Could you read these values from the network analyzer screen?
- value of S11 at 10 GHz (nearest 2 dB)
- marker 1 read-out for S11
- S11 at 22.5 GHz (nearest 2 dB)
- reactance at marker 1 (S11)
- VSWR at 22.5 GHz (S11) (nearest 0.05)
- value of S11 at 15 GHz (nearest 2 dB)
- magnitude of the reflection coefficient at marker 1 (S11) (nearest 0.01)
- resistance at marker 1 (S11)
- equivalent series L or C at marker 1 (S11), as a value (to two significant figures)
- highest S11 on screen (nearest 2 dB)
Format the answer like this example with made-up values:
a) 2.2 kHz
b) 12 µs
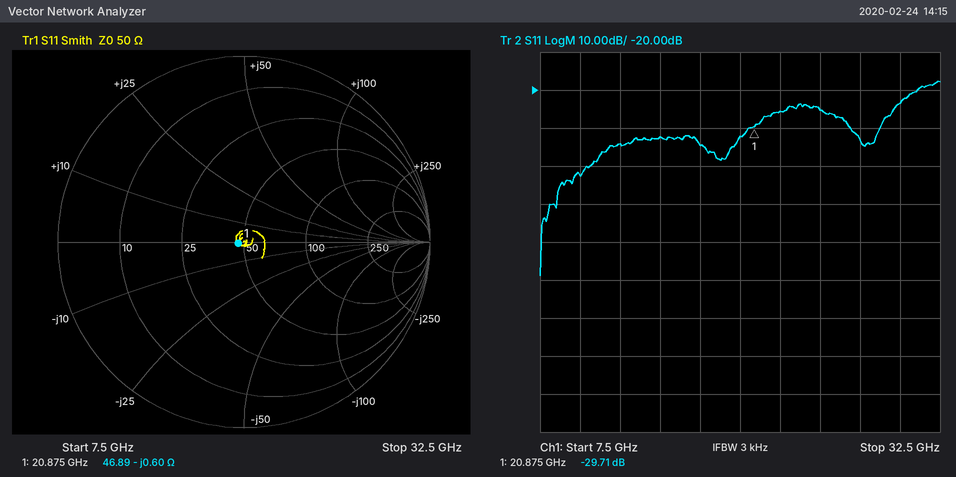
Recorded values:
a) -42 dB
b) -29.71 dB
c) -26 dB
d) -0.60 Ω
e) 1.10
f) -32 dB
g) 0.03
h) 46.89 Ω
i) 13 pF
j) -18 dB
